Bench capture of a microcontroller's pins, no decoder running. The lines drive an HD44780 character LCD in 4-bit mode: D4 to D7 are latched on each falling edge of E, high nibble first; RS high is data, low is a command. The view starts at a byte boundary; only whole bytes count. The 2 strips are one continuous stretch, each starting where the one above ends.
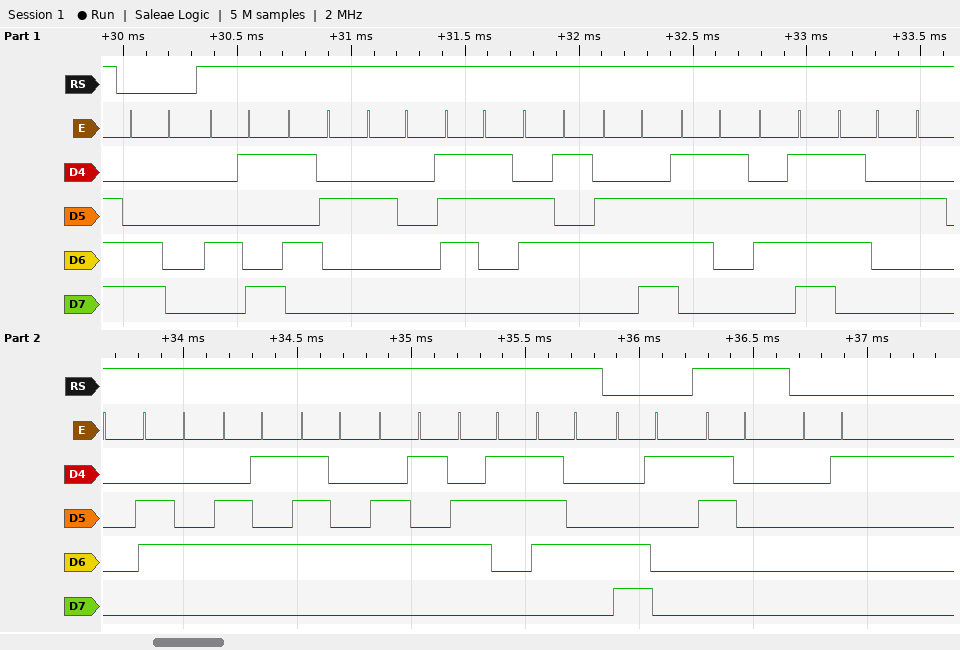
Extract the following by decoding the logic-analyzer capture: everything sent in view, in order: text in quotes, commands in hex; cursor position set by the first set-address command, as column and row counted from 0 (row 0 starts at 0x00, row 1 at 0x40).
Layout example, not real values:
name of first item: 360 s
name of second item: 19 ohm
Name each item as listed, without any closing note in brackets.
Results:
everything sent in view, in order: text in quotes, commands in hex: 0xC0 "IR sensor detect" 0xC1 "0" 0x01
cursor position set by the first set-address command, as column and row counted from 0: column 0, row 1
